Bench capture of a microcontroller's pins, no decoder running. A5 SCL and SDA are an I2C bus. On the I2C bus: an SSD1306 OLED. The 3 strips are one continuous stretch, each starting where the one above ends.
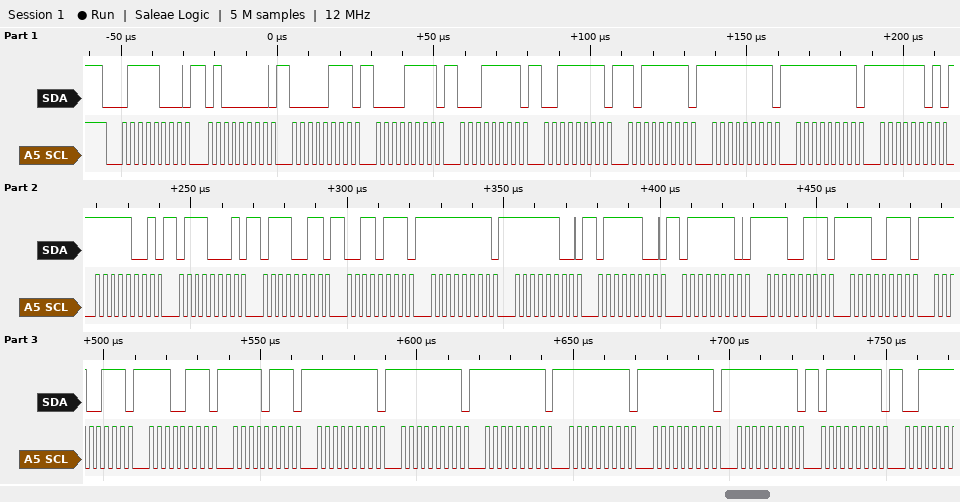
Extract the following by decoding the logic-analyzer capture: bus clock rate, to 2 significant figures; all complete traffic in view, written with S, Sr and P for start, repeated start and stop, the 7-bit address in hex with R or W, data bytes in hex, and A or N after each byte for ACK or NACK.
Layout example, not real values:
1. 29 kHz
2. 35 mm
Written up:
1. 400 kHz
2. S 3CW A 40 A 07 A 0F A 1F A 3F A BF A FF A FF A FD A F9 A 71 A 73 A 37 A FF A FC A 7C A 7E A E7 A E7 A E7 A E7 A F7 A FF A FF A FF A FF A FF A FF A 7F A
